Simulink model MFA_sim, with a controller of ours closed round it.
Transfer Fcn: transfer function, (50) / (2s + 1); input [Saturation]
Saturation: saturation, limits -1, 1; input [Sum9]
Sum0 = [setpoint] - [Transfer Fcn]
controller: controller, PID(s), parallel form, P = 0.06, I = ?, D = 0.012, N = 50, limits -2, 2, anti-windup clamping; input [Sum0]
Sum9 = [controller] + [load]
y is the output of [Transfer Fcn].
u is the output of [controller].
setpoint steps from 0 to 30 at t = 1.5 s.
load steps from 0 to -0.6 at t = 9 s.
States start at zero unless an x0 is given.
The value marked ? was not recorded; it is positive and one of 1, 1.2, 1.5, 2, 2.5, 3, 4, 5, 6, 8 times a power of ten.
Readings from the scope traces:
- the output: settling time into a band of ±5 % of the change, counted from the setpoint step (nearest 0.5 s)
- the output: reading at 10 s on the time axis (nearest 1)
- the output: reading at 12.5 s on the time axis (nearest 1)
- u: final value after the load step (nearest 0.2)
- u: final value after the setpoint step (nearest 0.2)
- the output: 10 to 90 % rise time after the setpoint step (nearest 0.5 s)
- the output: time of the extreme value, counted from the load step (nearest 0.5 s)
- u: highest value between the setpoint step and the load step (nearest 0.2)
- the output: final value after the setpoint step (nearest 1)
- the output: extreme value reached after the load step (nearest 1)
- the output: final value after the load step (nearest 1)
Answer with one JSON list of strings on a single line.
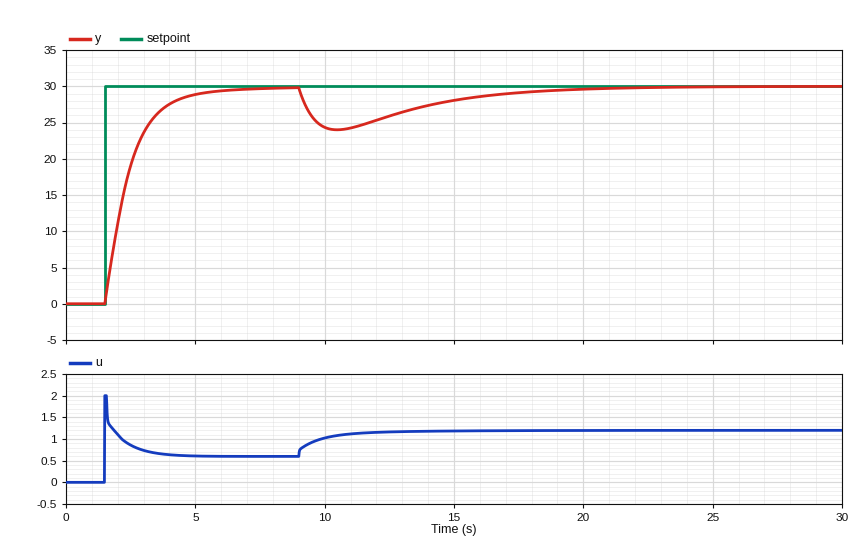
["3.0 s", "24", "26", "1.2", "0.6", "2.0 s", "1.5 s", "2.0", "30", "24", "30"]
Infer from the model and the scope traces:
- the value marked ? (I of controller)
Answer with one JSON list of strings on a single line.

["0.02"]
